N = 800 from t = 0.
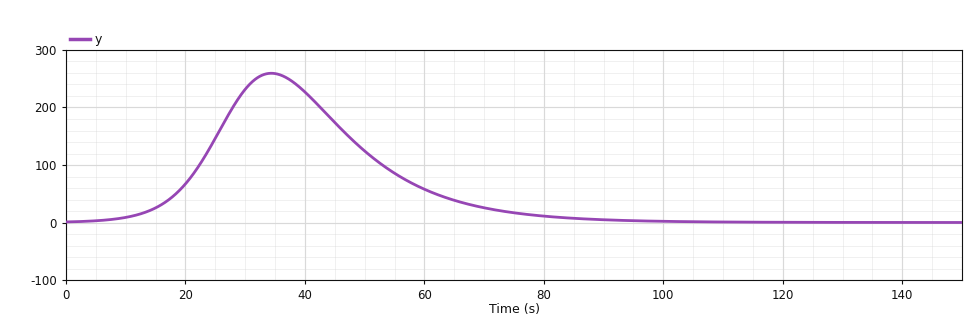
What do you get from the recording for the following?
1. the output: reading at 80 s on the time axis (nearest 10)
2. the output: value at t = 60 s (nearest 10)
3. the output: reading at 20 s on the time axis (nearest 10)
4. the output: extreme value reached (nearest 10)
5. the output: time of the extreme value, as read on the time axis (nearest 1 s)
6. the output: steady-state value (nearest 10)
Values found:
10
60
70
260
34 s
0
